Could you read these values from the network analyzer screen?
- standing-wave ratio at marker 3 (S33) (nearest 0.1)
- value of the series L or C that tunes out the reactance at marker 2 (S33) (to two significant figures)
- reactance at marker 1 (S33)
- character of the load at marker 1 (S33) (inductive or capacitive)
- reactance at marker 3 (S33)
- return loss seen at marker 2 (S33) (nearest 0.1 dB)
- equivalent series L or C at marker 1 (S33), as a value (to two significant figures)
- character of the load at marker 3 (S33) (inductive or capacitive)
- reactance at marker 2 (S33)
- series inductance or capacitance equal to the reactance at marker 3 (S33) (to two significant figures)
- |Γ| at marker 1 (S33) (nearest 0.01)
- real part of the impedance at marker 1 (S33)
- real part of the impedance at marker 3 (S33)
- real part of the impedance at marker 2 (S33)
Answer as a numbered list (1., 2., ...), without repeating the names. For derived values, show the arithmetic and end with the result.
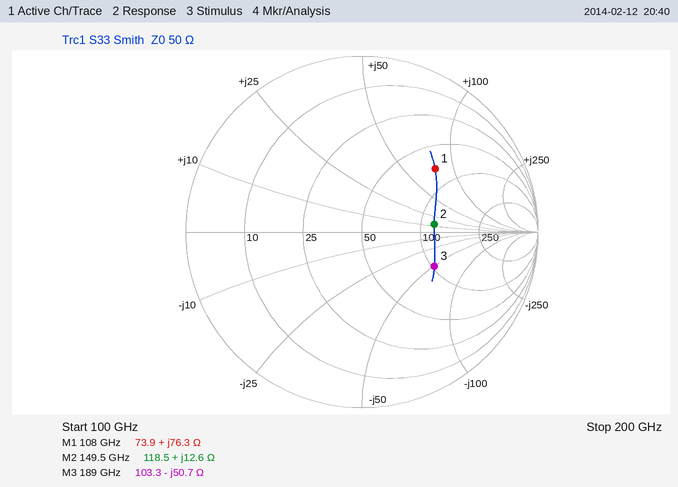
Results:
1. 2.7
2. C = 1/(2π × 149.5 GHz × 12.6 Ω) ≈ 84 fF
3. +76.3 Ω
4. inductive
5. -50.7 Ω
6. 7.7 dB
7. L = 76.3 Ω/(2π × 108 GHz) ≈ 112 pH, so 110 pH to two significant figures
8. capacitive
9. +12.6 Ω
10. C = 1/(2π × 189 GHz × 50.7 Ω) ≈ 17 fF
11. 0.55
12. 73.9 Ω
13. 103.3 Ω
14. 118.5 Ω
